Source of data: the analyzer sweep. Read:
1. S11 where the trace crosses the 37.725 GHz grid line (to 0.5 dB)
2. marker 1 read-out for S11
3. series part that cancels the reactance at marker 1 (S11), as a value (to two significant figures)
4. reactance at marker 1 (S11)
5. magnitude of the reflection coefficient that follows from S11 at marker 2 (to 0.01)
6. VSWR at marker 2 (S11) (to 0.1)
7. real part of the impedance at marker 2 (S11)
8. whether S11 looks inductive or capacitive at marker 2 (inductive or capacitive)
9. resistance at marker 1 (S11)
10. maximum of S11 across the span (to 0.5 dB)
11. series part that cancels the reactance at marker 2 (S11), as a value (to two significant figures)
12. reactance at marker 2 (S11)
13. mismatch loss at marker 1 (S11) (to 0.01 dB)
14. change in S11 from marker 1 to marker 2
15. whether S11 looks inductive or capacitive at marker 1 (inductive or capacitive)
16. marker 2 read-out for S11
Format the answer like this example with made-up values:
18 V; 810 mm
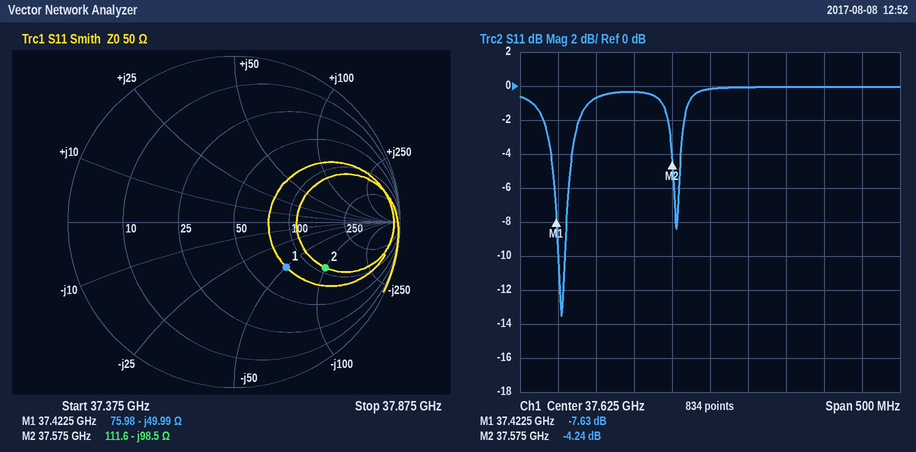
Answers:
0.0 dB; -7.63 dB; 210 pH; -49.99 Ω; 0.61; 4.2; 111.6 Ω; capacitive; 75.98 Ω; 0.0 dB; 420 pH; -98.5 Ω; 0.82 dB; 3.39 dB; capacitive; -4.24 dB
